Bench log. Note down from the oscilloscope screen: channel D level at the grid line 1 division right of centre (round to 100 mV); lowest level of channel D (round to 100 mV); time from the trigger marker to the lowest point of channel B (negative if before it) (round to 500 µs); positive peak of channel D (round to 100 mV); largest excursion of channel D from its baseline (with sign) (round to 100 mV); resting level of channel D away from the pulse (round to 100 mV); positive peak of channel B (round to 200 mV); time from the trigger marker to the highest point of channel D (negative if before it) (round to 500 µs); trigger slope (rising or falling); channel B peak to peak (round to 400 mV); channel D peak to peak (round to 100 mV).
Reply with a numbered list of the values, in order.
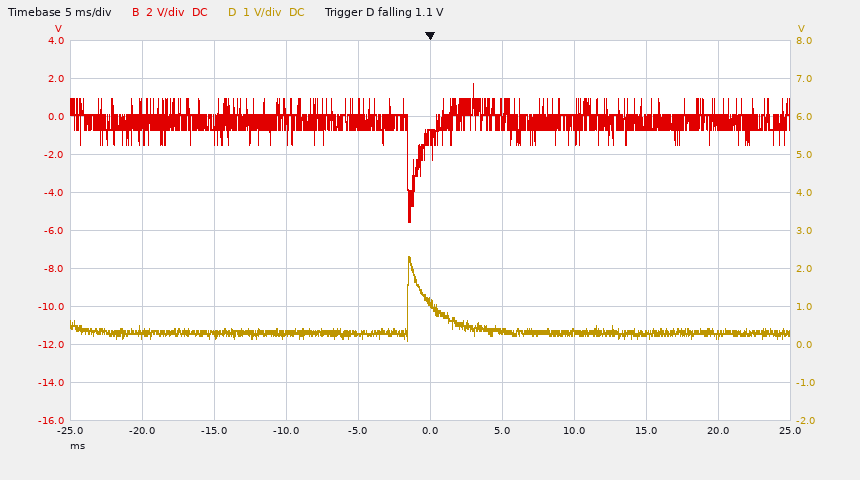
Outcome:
1. 400 mV
2. 100 mV
3. -1.5 ms
4. 2.3 V
5. +2.0 V
6. 300 mV
7. 1.8 V
8. -1.5 ms
9. falling
10. 7.2 V
11. 2.2 V
